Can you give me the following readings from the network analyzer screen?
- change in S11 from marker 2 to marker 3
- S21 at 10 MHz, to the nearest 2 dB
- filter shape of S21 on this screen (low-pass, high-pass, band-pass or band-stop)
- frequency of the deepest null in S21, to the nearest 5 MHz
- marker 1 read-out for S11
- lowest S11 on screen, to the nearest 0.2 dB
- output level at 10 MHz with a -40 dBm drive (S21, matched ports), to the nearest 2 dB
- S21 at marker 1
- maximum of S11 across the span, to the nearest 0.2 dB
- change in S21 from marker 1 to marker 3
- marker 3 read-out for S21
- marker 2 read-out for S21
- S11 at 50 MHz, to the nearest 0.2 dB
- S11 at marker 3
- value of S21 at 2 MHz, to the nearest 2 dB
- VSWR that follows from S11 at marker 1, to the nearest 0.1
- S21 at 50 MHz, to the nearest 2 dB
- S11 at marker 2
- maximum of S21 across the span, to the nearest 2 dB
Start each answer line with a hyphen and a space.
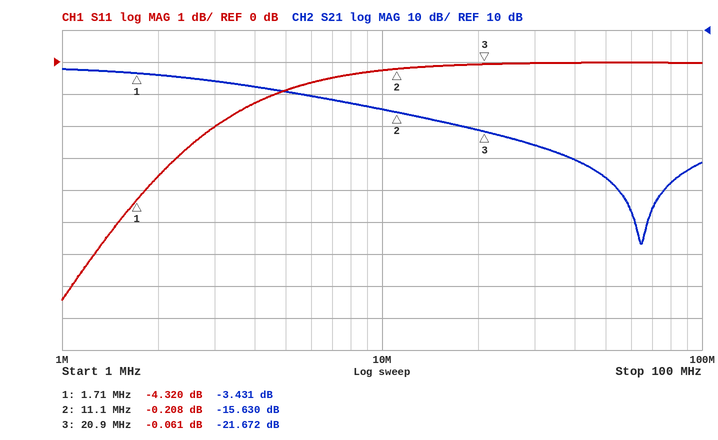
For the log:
- 0.147 dB
- -14 dB
- low-pass
- 65 MHz
- -4.320 dB
- -7.4 dB
- -54 dBm
- -3.431 dB
- 0.0 dB
- -18.241 dB
- -21.672 dB
- -15.630 dB
- 0.0 dB
- -0.061 dB
- -4 dB
- 4.1
- -36 dB
- -0.208 dB
- -2 dB
